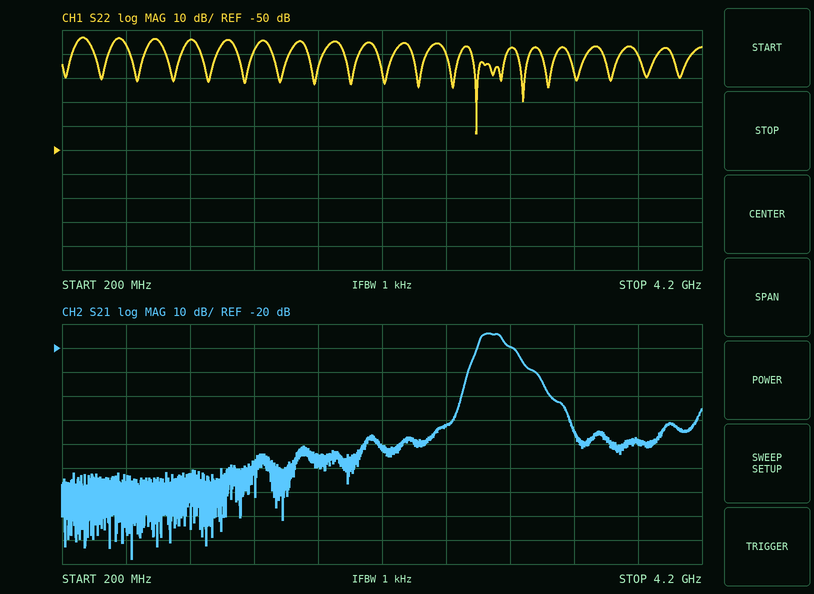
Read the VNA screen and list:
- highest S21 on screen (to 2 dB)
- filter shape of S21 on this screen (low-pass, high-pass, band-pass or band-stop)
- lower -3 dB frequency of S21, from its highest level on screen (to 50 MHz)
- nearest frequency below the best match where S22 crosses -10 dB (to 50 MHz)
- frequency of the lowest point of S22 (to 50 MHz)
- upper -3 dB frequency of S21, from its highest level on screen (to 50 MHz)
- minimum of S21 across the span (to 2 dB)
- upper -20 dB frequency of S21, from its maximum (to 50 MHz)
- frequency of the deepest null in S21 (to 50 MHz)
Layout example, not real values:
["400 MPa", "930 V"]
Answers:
["-14 dB", "band-pass", "2.80 GHz", "2.75 GHz", "2.80 GHz", "2.95 GHz", "-108 dB", "3.20 GHz", "650 MHz"]
